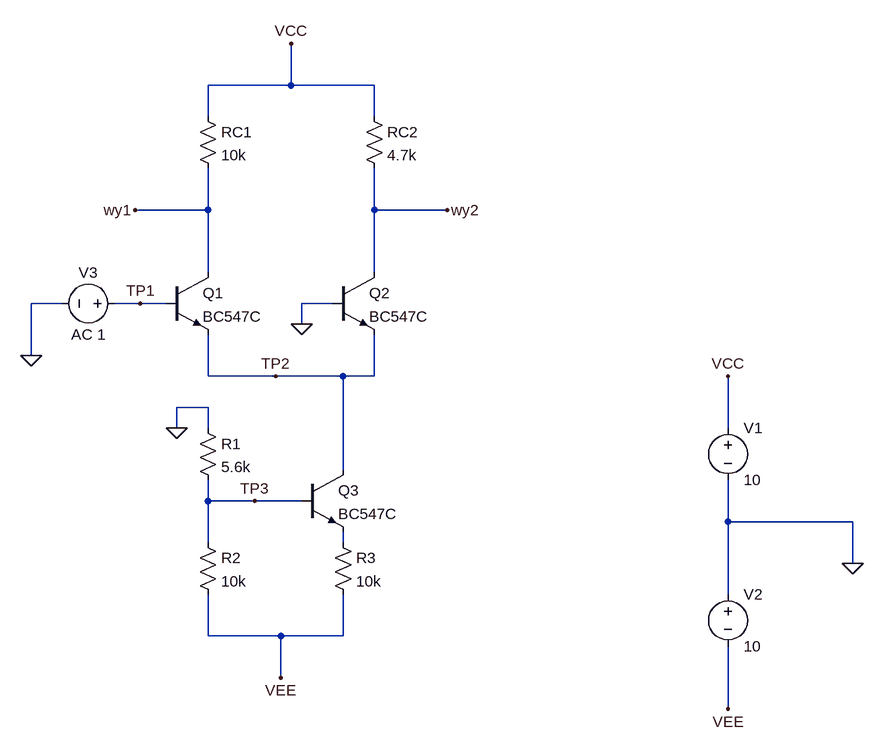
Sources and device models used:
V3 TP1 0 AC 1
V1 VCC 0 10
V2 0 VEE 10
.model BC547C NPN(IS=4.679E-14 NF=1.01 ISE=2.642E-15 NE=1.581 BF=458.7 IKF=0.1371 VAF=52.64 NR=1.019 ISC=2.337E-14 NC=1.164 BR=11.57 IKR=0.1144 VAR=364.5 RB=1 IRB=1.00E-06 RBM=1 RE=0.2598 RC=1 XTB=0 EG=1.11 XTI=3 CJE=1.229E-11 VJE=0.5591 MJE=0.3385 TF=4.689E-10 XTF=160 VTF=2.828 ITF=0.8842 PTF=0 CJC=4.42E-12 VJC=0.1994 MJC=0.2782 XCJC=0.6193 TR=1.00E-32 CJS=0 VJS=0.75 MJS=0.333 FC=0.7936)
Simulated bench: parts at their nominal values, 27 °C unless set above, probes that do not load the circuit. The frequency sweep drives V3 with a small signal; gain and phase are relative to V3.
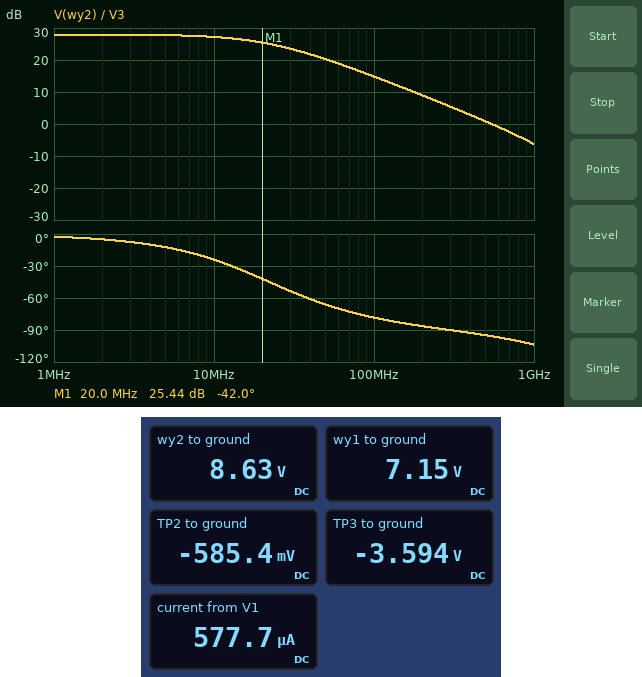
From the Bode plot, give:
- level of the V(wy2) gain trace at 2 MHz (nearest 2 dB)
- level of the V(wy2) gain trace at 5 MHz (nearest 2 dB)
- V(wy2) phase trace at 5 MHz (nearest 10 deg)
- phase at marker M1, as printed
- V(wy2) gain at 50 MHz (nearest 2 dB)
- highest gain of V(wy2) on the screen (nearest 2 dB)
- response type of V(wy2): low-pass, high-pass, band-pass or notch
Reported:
28 dB
28 dB
-10 deg
-42.0 deg
20 dB
28 dB
low-pass
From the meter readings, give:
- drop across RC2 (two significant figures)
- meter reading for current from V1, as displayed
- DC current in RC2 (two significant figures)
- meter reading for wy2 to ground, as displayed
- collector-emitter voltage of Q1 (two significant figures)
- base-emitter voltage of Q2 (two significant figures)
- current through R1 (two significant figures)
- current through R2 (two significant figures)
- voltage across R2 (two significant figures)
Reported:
1.4 V
577.7 µA
290 µA
8.63 V
7.7 V
590 mV
640 µA
640 µA
6.4 V
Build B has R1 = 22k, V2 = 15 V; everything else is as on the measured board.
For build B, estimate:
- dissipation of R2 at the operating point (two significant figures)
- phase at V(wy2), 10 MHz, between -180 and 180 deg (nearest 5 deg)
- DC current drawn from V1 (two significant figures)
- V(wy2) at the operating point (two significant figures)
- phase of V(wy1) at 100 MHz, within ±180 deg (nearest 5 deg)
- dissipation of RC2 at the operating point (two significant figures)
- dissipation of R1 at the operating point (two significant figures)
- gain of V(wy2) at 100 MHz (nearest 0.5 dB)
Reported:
2.2 mW
-25 deg
410 µA
9.0 V
80 deg
200 µW
4.8 mW
12.0 dB
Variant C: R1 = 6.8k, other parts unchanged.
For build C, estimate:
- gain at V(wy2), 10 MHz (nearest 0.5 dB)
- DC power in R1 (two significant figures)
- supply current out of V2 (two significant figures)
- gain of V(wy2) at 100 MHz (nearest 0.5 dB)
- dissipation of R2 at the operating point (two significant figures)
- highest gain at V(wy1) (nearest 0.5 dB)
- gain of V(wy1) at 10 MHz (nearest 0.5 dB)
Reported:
26.5 dB
2.4 mW
1.1 mA
14.0 dB
3.5 mW
34.0 dB
31.0 dB
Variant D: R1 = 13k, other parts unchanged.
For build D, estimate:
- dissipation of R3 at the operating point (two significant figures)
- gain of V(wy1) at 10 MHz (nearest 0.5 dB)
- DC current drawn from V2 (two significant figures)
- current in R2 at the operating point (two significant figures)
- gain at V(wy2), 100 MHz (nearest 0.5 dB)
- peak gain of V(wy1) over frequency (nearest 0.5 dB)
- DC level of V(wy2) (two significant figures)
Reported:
1.4 mW
28.0 dB
810 µA
430 µA
11.0 dB
31.0 dB
9.1 V
